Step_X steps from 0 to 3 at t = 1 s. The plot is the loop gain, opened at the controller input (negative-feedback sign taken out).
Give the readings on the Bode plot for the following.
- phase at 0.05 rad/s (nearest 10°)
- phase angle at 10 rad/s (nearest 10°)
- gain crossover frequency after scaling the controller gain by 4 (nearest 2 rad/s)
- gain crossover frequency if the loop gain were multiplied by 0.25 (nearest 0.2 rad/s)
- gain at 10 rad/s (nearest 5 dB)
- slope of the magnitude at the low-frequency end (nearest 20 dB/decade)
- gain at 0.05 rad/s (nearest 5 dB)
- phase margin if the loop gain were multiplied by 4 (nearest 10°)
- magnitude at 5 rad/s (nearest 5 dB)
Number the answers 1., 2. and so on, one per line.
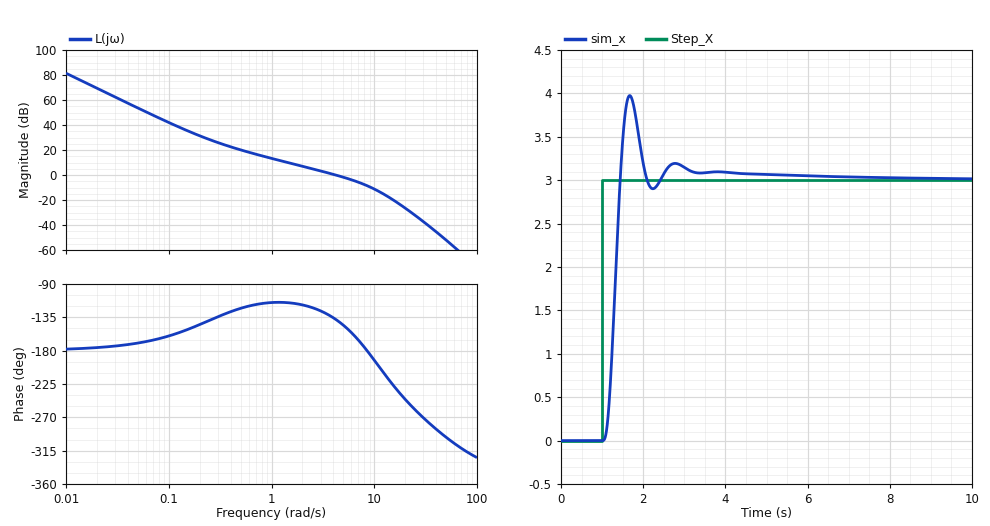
1. -170°
2. -190°
3. 10 rad/s
4. 1.2 rad/s
5. -10 dB
6. -40 dB/decade
7. 55 dB
8. -20°
9. 0 dB
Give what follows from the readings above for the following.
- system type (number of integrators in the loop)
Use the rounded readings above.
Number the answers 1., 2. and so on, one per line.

1. 2
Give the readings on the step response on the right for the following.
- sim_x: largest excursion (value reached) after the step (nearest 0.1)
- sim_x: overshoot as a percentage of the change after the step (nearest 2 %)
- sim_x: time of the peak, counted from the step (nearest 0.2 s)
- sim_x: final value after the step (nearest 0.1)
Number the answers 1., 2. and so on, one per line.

1. 4.0
2. 32 %
3. 0.6 s
4. 3.0
